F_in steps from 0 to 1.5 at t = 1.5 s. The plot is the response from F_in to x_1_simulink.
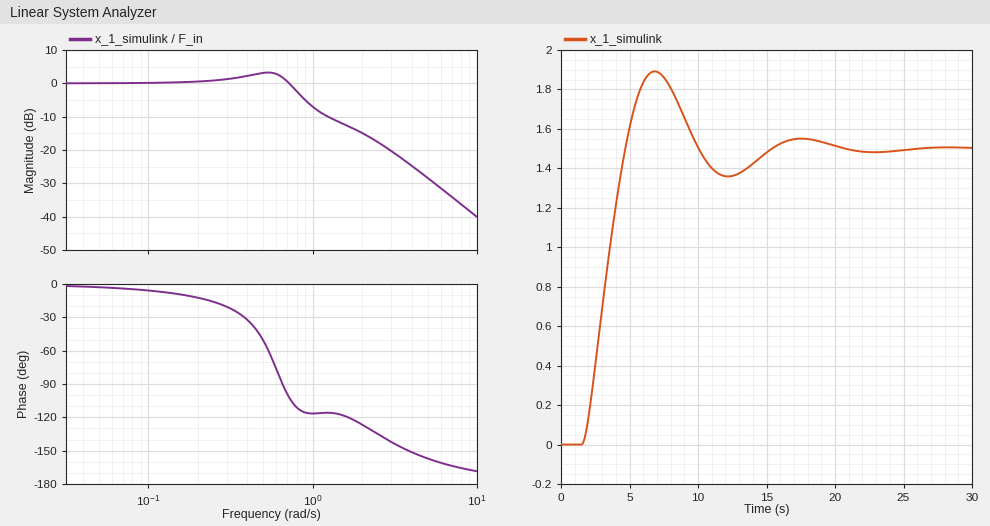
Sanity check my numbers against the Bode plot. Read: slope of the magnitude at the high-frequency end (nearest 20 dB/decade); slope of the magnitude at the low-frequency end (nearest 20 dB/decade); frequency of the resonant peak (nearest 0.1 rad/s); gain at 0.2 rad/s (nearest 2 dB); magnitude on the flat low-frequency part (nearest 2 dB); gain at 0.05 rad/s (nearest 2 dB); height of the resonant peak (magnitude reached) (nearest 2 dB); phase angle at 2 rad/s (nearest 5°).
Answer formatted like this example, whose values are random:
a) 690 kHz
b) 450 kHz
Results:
a) -40 dB/decade
b) 0 dB/decade
c) 0.5 rad/s
d) 0 dB
e) 0 dB
f) 0 dB
g) 4 dB
h) -125°
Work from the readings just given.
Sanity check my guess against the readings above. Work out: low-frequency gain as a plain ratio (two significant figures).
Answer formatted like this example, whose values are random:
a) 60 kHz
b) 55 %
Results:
a) 1.0
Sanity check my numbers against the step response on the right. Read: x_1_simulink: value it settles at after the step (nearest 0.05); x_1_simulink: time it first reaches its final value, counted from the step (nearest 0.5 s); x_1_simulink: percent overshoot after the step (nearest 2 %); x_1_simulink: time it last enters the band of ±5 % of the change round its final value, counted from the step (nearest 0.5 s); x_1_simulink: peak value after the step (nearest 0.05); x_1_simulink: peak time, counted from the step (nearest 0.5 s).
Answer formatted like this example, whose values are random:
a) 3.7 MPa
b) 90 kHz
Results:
a) 1.50
b) 3.0 s
c) 26 %
d) 12.5 s
e) 1.90
f) 5.5 s
